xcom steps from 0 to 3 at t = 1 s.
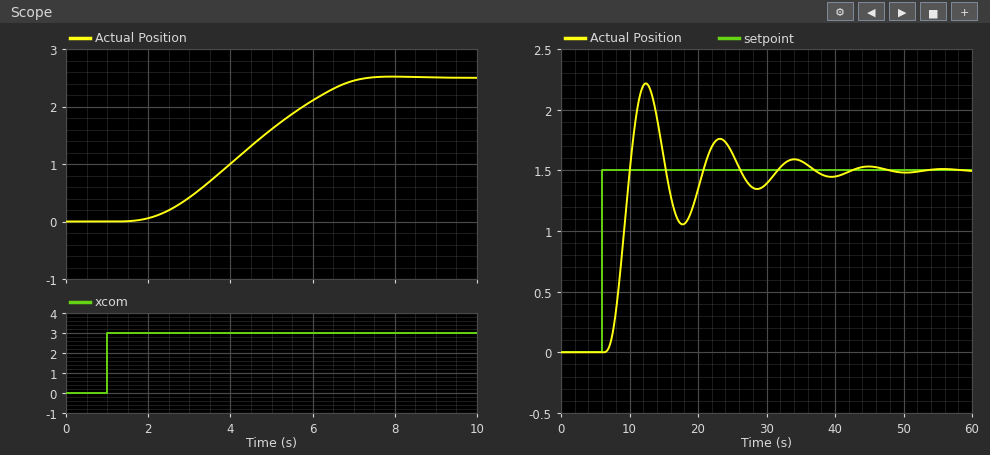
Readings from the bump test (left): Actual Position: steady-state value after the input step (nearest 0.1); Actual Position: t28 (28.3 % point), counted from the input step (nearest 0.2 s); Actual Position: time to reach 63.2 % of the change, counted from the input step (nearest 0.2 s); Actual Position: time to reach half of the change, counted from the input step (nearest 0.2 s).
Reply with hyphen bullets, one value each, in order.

- 2.5
- 2.6 s
- 4.0 s
- 3.4 s
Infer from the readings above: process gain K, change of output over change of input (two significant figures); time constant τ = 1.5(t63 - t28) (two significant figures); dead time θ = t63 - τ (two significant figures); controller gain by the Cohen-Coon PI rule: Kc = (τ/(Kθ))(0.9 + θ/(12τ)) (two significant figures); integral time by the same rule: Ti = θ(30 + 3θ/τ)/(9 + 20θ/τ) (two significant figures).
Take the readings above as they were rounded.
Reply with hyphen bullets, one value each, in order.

- 0.83
- 2.1 s
- 1.9 s
- 1.3
- 2.3 s
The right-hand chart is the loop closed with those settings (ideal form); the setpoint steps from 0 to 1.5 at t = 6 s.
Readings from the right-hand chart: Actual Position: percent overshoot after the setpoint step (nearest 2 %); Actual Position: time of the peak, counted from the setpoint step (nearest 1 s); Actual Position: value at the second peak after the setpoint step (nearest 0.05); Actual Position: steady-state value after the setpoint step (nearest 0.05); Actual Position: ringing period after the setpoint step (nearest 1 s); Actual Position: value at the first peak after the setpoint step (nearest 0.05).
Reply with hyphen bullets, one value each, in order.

- 48 %
- 6 s
- 1.75
- 1.50
- 11 s
- 2.20
